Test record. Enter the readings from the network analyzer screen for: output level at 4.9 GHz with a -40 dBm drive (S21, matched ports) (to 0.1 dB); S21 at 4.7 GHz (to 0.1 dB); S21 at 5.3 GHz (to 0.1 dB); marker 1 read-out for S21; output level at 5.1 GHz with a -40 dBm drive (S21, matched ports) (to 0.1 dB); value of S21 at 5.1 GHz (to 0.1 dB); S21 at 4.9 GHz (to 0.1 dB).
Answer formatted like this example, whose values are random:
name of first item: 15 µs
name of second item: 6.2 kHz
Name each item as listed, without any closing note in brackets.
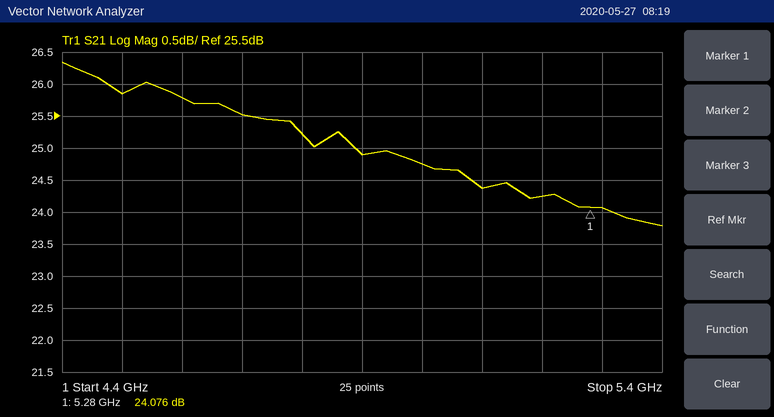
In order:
output level at 4.9 GHz with a -40 dBm drive (S21, matched ports): -15.1 dBm
S21 at 4.7 GHz: 25.5 dB
S21 at 5.3 GHz: 24.1 dB
marker 1 read-out for S21: 24.076 dB
output level at 5.1 GHz with a -40 dBm drive (S21, matched ports): -15.6 dBm
value of S21 at 5.1 GHz: 24.4 dB
S21 at 4.9 GHz: 24.9 dB
